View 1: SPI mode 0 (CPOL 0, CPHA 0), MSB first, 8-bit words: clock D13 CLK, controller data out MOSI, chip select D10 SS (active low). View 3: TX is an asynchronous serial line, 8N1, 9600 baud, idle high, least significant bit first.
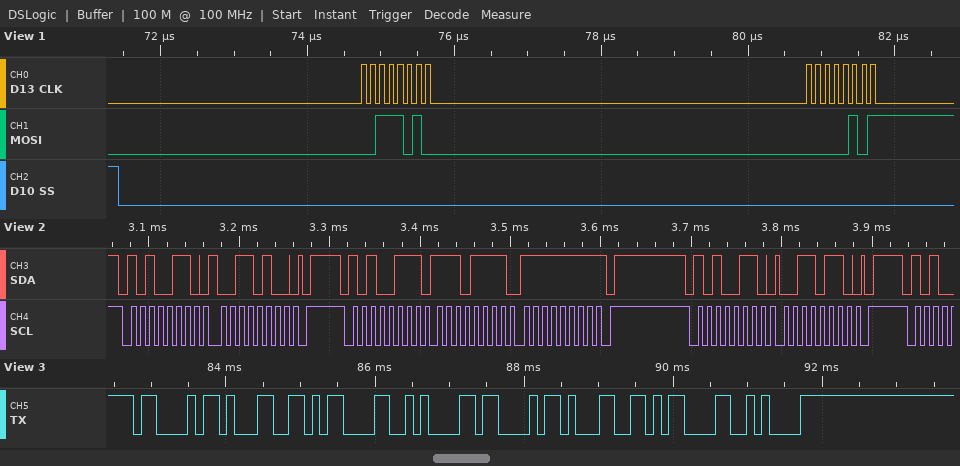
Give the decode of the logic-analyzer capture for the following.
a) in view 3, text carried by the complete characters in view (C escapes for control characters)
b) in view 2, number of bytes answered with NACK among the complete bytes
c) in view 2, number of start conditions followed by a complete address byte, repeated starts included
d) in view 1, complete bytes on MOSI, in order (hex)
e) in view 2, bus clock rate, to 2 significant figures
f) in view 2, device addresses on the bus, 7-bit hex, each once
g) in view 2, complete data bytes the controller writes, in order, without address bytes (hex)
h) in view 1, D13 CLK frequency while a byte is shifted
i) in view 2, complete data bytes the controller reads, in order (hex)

"C1\r\nC1\r\n"
1
3
3A 05
100 kHz
0x53
34 36
8 MHz
EF FF
